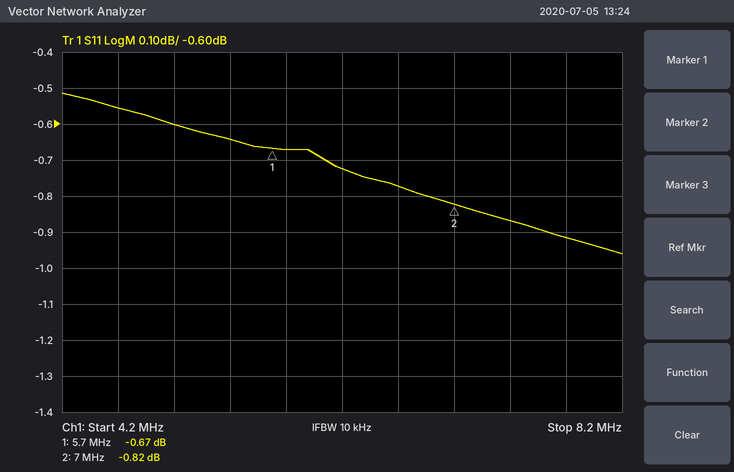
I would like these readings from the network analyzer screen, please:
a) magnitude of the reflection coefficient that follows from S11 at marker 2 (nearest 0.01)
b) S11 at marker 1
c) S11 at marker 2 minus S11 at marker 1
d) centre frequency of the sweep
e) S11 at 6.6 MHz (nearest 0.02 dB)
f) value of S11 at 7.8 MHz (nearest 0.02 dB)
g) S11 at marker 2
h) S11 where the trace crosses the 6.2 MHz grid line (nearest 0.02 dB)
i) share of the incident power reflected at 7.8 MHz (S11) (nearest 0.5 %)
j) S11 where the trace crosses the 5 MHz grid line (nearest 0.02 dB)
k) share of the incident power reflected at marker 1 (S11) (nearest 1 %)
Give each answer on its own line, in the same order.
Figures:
0.91
-0.67 dB
-0.15 dB
6.2 MHz
-0.78 dB
-0.92 dB
-0.82 dB
-0.72 dB
81.0 %
-0.60 dB
86 %
